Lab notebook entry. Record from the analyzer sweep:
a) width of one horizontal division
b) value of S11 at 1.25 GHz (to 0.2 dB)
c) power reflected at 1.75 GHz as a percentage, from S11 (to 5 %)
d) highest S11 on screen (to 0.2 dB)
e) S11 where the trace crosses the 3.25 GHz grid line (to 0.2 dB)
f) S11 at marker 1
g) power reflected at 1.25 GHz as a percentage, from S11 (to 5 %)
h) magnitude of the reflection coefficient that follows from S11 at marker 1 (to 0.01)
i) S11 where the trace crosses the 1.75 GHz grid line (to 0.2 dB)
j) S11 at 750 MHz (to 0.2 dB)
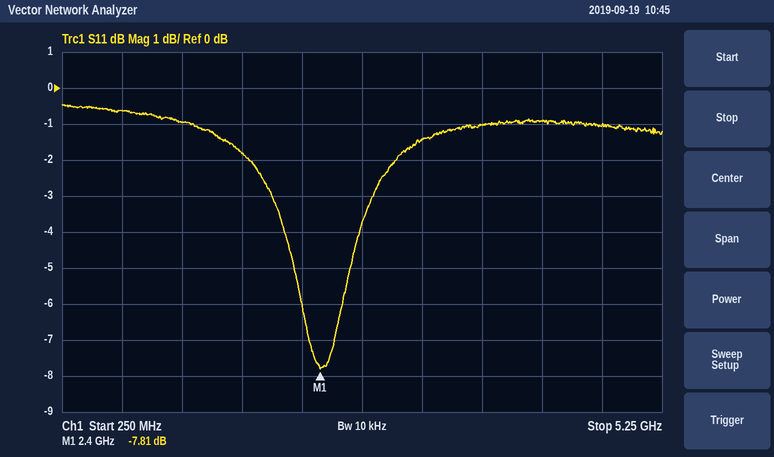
500 MHz
-1.0 dB
65 %
-0.4 dB
-1.4 dB
-7.81 dB
80 %
0.41
-1.8 dB
-0.6 dB
